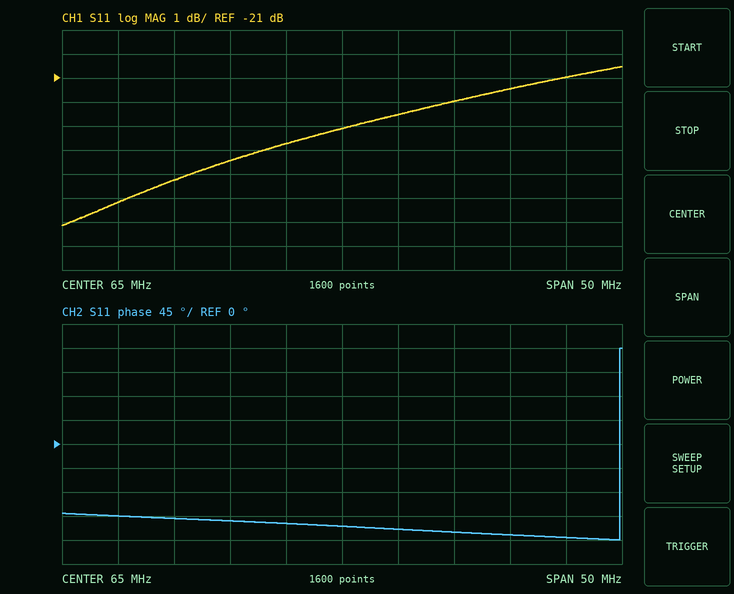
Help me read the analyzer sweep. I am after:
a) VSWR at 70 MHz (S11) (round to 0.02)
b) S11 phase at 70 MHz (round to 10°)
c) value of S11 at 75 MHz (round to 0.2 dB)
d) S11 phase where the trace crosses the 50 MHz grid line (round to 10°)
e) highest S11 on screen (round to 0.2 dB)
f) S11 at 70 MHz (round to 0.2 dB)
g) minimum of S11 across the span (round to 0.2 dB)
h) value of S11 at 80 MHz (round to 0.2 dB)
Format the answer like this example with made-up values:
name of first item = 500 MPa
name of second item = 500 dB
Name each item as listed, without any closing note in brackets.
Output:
VSWR at 70 MHz (S11) = 1.16
S11 phase at 70 MHz = -160°
value of S11 at 75 MHz = -22.0 dB
S11 phase where the trace crosses the 50 MHz grid line = -140°
highest S11 on screen = -20.6 dB
S11 at 70 MHz = -22.6 dB
minimum of S11 across the span = -27.2 dB
value of S11 at 80 MHz = -21.4 dB
